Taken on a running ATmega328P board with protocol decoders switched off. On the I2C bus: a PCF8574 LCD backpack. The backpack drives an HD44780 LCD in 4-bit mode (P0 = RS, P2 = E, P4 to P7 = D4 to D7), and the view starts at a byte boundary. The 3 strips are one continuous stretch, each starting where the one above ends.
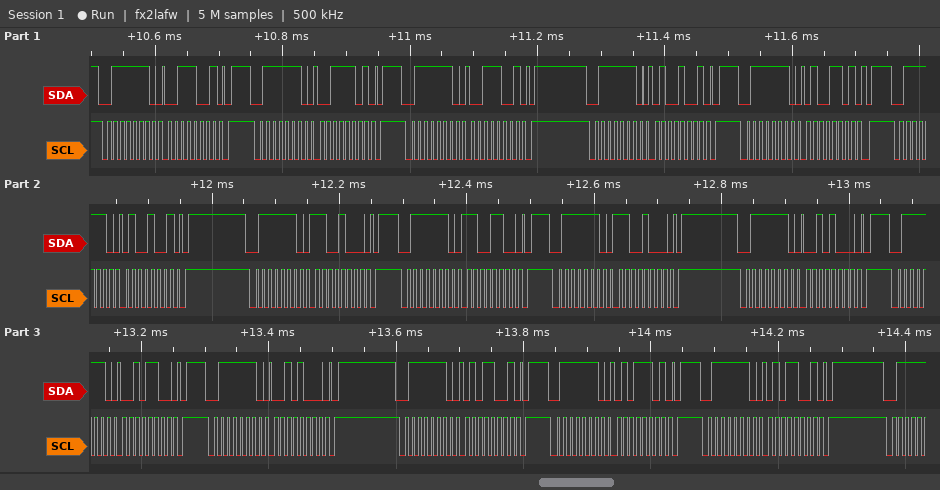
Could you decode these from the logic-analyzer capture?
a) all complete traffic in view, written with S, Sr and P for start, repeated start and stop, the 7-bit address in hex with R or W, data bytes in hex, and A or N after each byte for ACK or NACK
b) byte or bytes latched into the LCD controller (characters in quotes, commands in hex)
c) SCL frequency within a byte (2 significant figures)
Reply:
S 3FW A 39 A P S 3FW A 3D A P S 3FW A 39 A P S 3FW A 49 A P S 3FW A 4D A P S 3FW A 49 A P S 3FW A C8 A P S 3FW A CC A P S 3FW A C8 A P S 3FW A 28 A P S 3FW A 2C A P S 3FW A 28 A P S 3FW A 59 A P S 3FW A 5D A P S 3FW A 59 A P
'4' 0xC2
100 kHz
